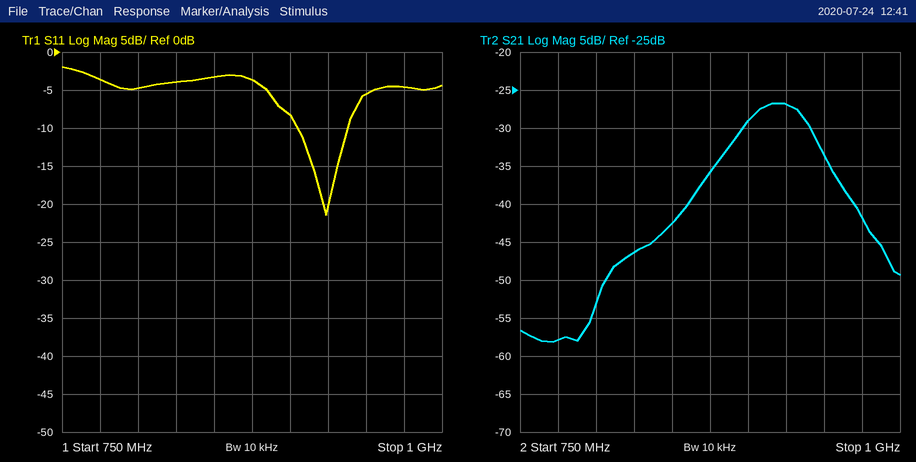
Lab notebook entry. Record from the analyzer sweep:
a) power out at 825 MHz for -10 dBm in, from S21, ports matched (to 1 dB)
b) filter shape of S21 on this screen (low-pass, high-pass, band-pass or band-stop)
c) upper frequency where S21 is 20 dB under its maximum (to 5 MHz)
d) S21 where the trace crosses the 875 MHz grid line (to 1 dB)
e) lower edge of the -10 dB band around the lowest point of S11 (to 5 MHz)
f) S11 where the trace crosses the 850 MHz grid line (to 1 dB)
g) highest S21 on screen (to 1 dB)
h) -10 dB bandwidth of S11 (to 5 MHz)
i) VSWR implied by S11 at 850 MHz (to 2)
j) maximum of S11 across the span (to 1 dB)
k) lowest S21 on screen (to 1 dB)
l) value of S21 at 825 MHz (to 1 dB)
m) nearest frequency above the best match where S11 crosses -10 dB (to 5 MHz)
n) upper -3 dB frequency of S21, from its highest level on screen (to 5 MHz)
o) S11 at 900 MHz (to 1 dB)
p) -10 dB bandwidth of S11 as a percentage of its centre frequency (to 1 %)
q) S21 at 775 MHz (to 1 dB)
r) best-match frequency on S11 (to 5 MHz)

-56 dBm
band-pass
990 MHz
-36 dB
905 MHz
-3 dB
-27 dB
35 MHz
6
-2 dB
-58 dB
-46 dB
940 MHz
940 MHz
-8 dB
4 %
-58 dB
925 MHz
